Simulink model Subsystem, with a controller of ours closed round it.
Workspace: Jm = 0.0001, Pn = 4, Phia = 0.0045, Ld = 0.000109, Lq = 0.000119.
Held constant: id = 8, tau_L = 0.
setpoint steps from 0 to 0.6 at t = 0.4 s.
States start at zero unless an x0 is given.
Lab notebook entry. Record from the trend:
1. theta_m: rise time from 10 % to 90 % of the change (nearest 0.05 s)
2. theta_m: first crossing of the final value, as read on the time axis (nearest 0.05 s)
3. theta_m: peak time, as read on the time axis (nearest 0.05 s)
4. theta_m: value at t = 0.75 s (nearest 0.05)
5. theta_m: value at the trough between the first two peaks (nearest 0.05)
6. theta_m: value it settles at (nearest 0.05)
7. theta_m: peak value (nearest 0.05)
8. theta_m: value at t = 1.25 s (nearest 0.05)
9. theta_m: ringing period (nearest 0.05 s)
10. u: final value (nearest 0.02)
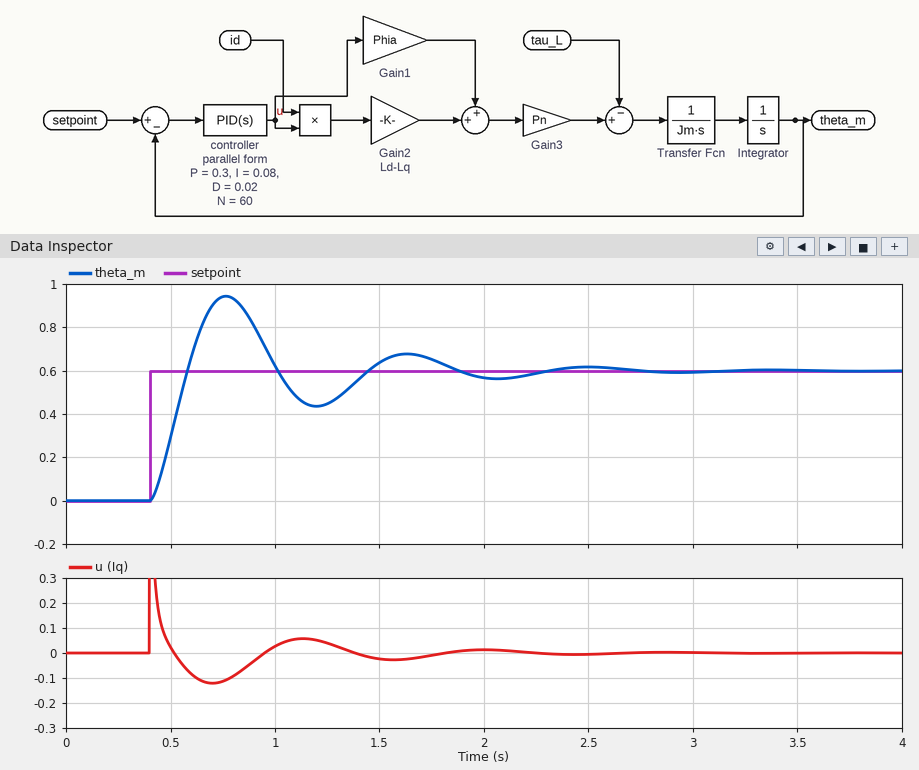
0.15 s
0.60 s
0.75 s
0.95
0.45
0.60
0.95
0.45
0.85 s
0.00
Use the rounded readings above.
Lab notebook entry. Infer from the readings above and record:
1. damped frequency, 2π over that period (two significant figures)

7.4 rad/s
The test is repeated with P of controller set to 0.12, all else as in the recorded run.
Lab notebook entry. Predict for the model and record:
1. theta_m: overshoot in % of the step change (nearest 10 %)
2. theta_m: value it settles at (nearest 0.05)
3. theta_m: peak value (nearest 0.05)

50 %
0.60
0.90
